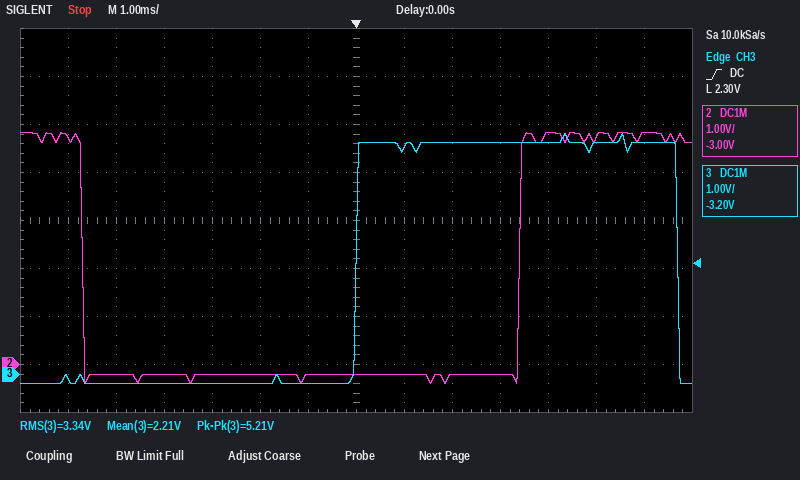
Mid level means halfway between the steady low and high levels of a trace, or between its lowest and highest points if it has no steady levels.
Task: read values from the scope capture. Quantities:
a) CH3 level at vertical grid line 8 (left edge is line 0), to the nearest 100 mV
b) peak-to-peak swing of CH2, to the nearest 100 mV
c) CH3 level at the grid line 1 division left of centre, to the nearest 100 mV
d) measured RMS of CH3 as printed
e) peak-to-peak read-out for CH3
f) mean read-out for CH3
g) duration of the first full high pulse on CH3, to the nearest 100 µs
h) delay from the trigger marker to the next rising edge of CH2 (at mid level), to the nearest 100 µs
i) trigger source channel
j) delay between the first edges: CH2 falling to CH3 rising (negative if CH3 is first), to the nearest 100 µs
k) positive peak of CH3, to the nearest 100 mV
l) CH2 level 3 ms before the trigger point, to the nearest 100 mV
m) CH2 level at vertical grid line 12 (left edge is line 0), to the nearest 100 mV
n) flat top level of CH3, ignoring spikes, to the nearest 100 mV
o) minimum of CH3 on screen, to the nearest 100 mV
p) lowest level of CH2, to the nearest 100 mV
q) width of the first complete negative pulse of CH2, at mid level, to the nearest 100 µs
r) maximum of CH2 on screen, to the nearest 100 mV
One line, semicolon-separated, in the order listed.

4.7 V; 5.2 V; -200 mV; 3.34 V; 5.21 V; 2.21 V; 6.7 ms; 3.4 ms; CH3; +5.7 ms; 5.0 V; -200 mV; 4.7 V; 4.8 V; -200 mV; -400 mV; 9.1 ms; 4.8 V
